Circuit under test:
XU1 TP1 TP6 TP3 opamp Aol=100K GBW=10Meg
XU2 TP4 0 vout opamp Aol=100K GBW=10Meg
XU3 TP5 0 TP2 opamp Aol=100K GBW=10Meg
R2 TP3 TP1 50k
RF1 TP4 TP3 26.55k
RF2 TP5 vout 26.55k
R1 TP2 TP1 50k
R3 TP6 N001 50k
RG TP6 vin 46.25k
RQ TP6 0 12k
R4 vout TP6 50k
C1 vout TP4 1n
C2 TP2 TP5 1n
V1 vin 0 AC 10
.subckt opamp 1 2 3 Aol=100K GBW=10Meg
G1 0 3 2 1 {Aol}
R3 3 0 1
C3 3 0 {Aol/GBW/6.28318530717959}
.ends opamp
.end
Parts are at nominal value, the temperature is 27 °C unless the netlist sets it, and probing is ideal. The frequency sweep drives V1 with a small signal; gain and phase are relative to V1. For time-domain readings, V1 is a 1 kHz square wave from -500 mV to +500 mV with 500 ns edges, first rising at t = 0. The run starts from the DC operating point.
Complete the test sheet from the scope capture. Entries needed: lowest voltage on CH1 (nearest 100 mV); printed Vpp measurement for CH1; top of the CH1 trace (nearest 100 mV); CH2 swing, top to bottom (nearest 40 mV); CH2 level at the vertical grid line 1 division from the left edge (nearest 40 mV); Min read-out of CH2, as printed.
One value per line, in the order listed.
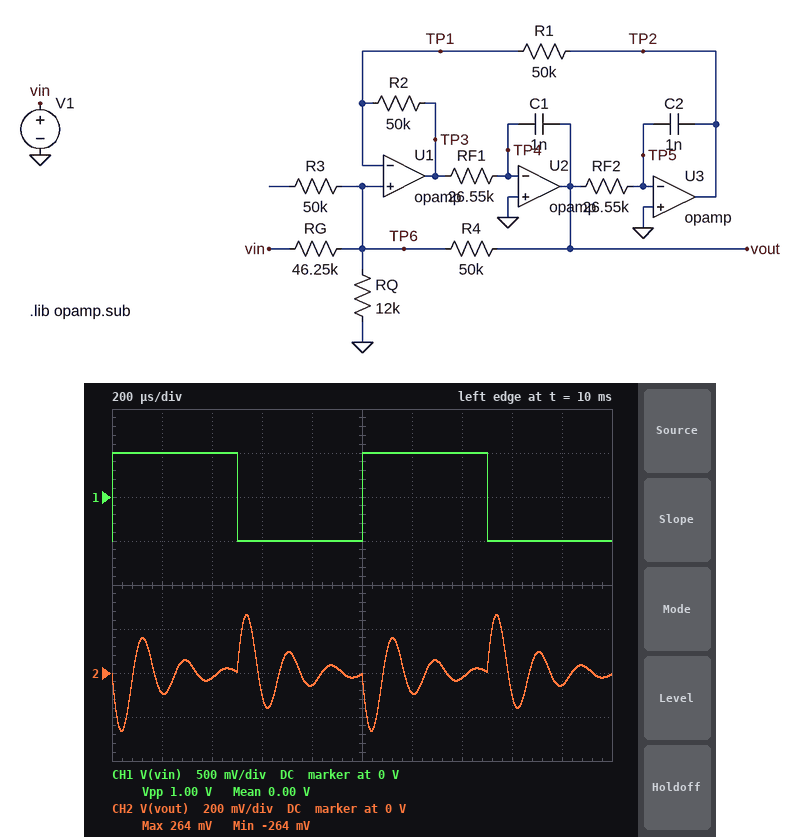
-500 mV
1.00 V
500 mV
520 mV
-80 mV
-264 mV
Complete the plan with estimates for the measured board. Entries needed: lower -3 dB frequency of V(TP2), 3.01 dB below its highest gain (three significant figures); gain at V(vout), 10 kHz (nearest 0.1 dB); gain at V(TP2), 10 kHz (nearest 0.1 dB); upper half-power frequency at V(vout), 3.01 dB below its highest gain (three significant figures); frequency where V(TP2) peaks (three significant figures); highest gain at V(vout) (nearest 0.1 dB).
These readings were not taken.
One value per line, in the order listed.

4.78 kHz
-10.2 dB
-14.6 dB
7.02 kHz
5.84 kHz
0.7 dB
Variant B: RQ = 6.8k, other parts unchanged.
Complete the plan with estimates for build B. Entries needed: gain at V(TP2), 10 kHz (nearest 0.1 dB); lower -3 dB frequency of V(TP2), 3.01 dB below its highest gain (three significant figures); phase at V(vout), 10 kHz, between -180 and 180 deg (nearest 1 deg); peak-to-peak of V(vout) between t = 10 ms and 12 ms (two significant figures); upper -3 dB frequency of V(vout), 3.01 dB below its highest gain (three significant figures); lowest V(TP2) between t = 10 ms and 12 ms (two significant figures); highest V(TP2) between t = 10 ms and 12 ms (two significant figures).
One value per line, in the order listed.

-18.0 dB
5.26 kHz
101 deg
350 mV
6.65 kHz
-260 mV
260 mV
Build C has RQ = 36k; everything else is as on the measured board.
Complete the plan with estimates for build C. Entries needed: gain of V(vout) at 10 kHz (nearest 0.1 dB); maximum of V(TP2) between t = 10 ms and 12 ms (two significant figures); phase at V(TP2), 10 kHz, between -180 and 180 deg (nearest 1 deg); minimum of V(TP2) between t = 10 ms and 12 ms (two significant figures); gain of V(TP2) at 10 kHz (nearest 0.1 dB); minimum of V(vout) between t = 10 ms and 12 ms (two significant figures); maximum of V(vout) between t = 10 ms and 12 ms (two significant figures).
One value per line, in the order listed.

-5.8 dB
550 mV
-152 deg
-550 mV
-10.2 dB
-420 mV
420 mV
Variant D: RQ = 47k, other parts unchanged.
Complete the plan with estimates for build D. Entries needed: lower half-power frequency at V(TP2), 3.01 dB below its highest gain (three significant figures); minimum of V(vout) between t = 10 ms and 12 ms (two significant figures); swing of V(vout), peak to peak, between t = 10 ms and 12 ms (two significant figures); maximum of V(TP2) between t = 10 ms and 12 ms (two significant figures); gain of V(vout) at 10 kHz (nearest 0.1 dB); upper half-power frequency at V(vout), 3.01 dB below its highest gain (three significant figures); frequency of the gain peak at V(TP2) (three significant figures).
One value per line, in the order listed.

2.67 kHz
-450 mV
910 mV
580 mV
-5.1 dB
8.19 kHz
5.36 kHz
